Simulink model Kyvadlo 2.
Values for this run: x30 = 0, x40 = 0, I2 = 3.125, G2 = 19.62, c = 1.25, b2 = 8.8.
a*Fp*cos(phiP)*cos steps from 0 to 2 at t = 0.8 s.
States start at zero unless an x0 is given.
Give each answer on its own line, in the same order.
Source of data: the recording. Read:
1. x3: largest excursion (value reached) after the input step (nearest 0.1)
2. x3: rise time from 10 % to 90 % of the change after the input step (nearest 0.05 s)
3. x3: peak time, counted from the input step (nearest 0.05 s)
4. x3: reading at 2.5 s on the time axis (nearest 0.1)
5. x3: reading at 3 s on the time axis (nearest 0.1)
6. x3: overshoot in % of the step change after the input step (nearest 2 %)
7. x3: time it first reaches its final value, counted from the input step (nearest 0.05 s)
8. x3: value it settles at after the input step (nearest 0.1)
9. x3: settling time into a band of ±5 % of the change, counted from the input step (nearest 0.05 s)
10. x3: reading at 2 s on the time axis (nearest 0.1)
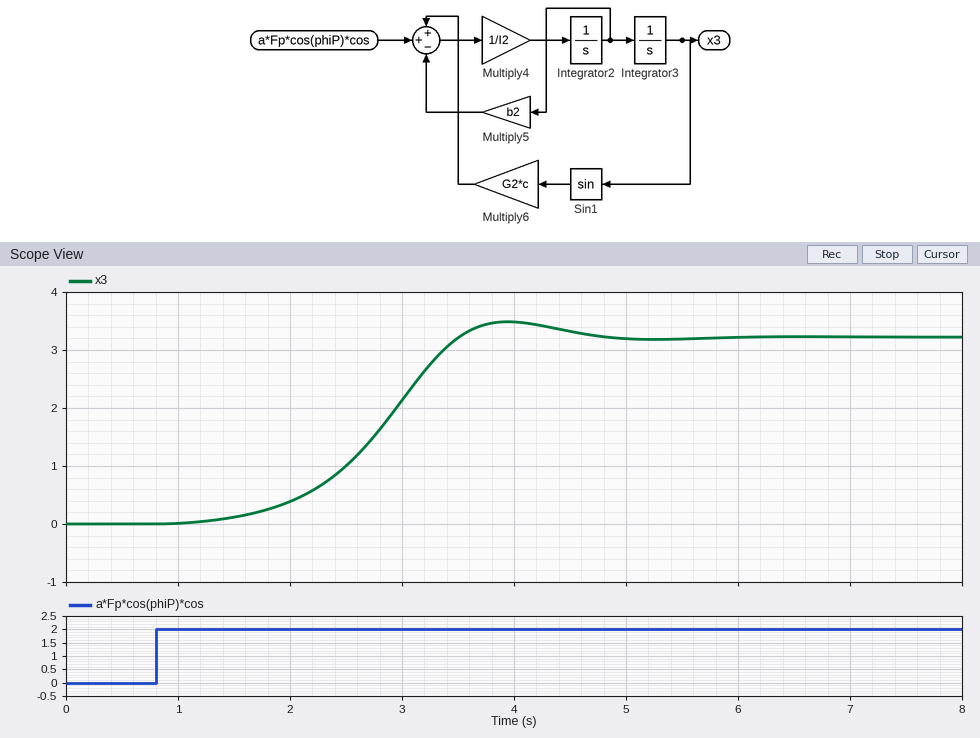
3.5
1.40 s
3.15 s
1.0
2.1
8 %
2.70 s
3.2
3.55 s
0.4
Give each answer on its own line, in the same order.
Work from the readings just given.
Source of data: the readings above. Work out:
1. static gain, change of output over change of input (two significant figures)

1.6
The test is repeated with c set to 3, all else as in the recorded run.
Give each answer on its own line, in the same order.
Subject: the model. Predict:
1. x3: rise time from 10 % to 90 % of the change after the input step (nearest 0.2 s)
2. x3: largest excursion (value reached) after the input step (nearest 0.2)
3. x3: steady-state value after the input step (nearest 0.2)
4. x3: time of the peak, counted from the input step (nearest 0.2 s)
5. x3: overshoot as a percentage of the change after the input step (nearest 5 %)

0.8 s
3.8
3.2
2.0 s
20 %
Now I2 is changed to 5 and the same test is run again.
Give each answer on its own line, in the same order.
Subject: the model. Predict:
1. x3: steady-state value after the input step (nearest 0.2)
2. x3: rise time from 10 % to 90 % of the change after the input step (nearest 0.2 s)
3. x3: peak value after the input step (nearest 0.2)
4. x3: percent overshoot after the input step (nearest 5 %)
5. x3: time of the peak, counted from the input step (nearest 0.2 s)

3.2
1.6 s
3.6
15 %
3.6 s
